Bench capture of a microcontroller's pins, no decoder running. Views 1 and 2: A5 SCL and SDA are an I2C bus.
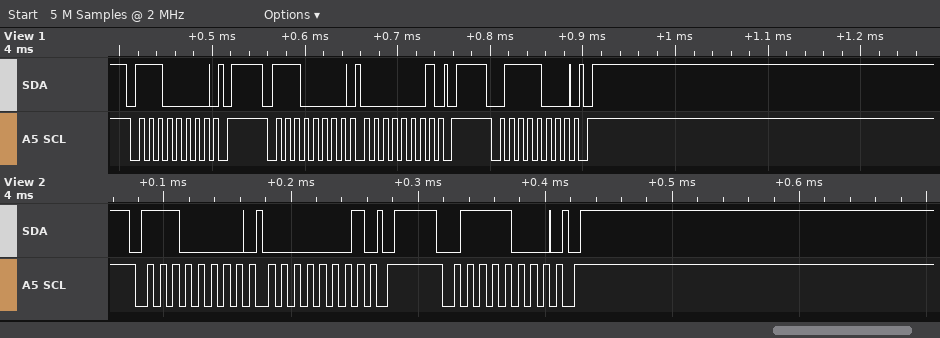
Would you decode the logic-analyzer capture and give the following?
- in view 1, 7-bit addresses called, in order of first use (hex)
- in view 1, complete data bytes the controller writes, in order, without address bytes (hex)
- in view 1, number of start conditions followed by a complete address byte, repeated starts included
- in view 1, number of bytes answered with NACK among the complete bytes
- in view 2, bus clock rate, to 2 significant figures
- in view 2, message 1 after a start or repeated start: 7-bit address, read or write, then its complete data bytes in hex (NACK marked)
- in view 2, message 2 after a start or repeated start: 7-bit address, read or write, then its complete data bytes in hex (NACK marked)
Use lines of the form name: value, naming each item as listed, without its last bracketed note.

in view 1, 7-bit addresses called, in order of first use: 0x70 0x3C
in view 1, complete data bytes the controller writes, in order, without address bytes: 01
in view 1, number of start conditions followed by a complete address byte, repeated starts included: 3
in view 1, number of bytes answered with NACK among the complete bytes: 0
in view 2, bus clock rate, to 2 significant figures: 100 kHz
in view 2, message 1 after a start or repeated start: 7-bit address, read or write, then its complete data bytes in hex: 0x70 write: 01
in view 2, message 2 after a start or repeated start: 7-bit address, read or write, then its complete data bytes in hex: 0x3C write
